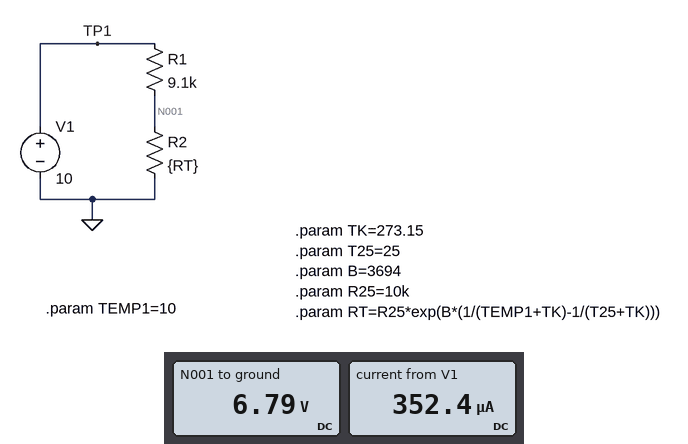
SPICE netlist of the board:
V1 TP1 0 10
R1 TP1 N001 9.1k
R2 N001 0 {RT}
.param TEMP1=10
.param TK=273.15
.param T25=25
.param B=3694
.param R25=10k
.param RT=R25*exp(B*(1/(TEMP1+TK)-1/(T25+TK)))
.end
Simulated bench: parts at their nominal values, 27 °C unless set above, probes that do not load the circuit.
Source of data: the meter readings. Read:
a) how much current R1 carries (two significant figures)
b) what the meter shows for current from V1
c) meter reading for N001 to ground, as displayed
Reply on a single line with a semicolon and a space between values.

350 µA; 352.4 µA; 6.79 V
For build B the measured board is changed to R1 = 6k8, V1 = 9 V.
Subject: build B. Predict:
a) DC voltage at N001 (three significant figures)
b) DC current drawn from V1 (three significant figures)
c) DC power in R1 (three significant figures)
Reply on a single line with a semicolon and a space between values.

6.65 V; 345 µA; 810 µW
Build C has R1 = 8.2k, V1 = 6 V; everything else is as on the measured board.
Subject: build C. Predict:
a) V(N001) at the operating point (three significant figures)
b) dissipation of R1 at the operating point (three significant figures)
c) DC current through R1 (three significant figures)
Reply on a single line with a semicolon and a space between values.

4.21 V; 391 µW; 218 µA
